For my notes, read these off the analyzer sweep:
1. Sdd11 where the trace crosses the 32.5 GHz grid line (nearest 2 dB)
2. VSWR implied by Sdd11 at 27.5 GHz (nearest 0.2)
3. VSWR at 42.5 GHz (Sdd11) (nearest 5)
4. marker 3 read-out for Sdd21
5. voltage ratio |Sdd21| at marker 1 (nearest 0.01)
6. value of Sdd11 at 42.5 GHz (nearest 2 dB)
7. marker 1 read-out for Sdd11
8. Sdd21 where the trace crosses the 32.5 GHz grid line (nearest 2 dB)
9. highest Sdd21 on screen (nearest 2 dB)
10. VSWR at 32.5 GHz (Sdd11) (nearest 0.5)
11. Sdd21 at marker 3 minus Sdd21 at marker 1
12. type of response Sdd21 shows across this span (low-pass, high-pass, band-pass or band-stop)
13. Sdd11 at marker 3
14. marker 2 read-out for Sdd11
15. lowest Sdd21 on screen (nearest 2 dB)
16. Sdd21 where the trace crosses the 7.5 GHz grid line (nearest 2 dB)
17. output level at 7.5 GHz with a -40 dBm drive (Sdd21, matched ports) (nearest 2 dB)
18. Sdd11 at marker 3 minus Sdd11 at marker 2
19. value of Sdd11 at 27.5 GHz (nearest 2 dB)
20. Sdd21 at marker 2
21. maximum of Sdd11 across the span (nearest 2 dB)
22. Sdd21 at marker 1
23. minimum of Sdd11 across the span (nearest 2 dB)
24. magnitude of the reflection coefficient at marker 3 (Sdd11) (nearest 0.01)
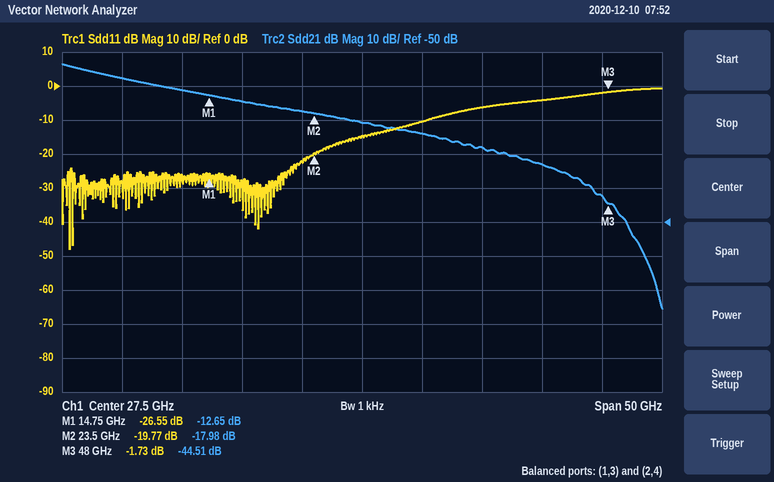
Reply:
-10 dB
1.4
5
-44.51 dB
0.23
-4 dB
-26.55 dB
-24 dB
-4 dB
2.0
-31.86 dB
low-pass
-1.73 dB
-19.77 dB
-76 dB
-8 dB
-48 dBm
18.04 dB
-14 dB
-17.98 dB
0 dB
-12.65 dB
-48 dB
0.82
